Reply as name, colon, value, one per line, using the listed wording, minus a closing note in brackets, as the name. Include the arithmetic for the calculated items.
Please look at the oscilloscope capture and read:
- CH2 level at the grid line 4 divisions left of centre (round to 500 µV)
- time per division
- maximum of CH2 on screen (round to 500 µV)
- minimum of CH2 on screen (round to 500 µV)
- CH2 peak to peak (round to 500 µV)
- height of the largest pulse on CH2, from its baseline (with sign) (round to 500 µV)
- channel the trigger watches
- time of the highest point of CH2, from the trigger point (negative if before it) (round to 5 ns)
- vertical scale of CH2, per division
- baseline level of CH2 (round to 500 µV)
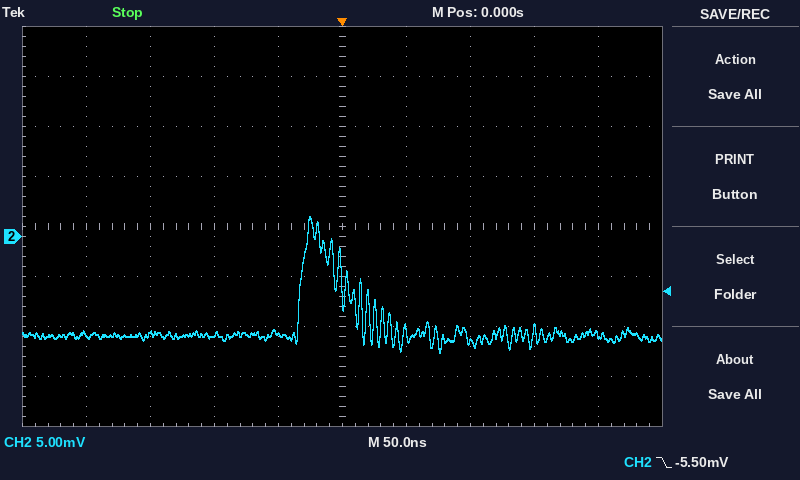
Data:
CH2 level at the grid line 4 divisions left of centre: -10.0 mV
time per division: 50 ns
maximum of CH2 on screen: 2.0 mV
minimum of CH2 on screen: -11.5 mV
CH2 peak to peak: 2.0 mV − (-11.5 mV) = 13.5 mV
height of the largest pulse on CH2, from its baseline (with sign): 2.0 mV − (-10.0 mV) = +12.0 mV
channel the trigger watches: CH2
time of the highest point of CH2, from the trigger point (negative if before it): -25 ns
vertical scale of CH2, per division: 5 mV
baseline level of CH2: -10.0 mV
